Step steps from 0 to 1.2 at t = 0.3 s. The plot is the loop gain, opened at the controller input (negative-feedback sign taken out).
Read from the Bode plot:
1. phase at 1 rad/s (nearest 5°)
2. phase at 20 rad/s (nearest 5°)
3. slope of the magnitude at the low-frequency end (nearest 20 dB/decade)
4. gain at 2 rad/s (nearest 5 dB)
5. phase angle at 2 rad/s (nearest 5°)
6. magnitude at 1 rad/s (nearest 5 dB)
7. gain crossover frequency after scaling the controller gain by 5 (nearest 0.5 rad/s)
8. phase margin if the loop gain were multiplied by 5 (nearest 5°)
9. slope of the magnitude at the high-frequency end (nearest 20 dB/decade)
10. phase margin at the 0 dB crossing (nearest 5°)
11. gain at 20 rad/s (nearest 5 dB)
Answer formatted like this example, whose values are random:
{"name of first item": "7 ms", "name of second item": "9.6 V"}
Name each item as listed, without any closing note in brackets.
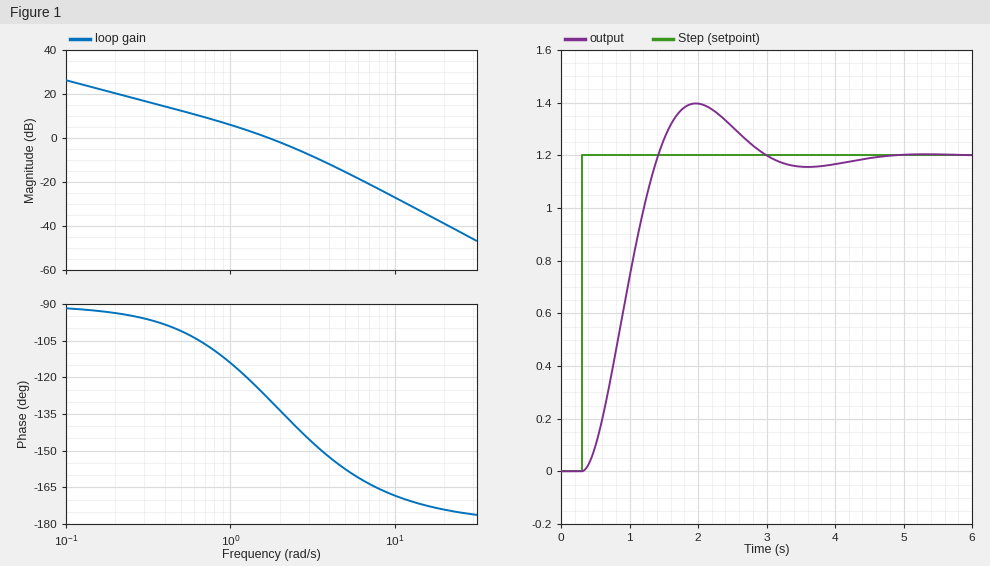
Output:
{"phase at 1 rad/s": "-115°", "phase at 20 rad/s": "-175°", "slope of the magnitude at the low-frequency end": "-20 dB/decade", "gain at 2 rad/s": "0 dB", "phase angle at 2 rad/s": "-135°", "magnitude at 1 rad/s": "5 dB", "gain crossover frequency after scaling the controller gain by 5": "4.5 rad/s", "phase margin if the loop gain were multiplied by 5": "25°", "slope of the magnitude at the high-frequency end": "-40 dB/decade", "phase margin at the 0 dB crossing": "50°", "gain at 20 rad/s": "-40 dB"}
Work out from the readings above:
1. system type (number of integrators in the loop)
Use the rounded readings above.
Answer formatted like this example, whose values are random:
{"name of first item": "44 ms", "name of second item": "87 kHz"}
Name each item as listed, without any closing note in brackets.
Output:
{"system type": "1"}
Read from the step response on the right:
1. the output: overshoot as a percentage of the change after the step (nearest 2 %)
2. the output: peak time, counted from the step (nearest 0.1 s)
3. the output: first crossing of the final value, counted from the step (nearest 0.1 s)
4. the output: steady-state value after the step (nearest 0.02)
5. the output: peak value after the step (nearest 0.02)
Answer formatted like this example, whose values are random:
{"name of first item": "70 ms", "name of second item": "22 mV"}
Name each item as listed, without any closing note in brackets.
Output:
{"the output: overshoot as a percentage of the change after the step": "16 %", "the output: peak time, counted from the step": "1.7 s", "the output: first crossing of the final value, counted from the step": "1.1 s", "the output: steady-state value after the step": "1.20", "the output: peak value after the step": "1.40"}
